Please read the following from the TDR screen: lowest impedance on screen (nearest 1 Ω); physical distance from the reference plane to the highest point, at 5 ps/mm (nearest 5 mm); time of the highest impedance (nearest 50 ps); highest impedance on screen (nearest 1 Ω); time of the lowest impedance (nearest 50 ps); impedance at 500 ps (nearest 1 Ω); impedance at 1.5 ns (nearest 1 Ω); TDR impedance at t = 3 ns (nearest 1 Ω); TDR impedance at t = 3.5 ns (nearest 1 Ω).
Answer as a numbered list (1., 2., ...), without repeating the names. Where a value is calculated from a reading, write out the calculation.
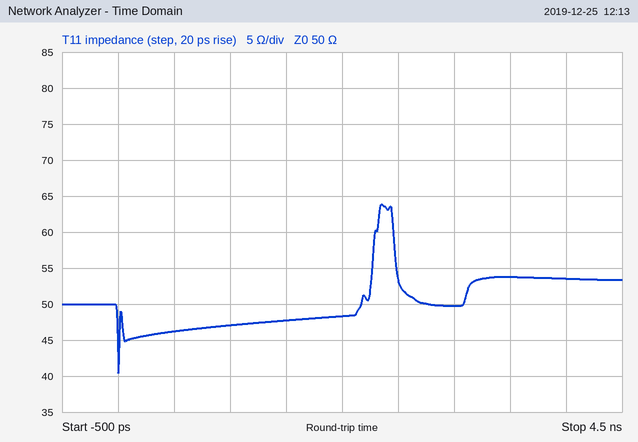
1. 40 Ω
2. 2.35 ns / 2 / 5 ps/mm ≈ 235 mm
3. 2.35 ns
4. 64 Ω
5. 0 ps
6. 46 Ω
7. 48 Ω
8. 50 Ω
9. 54 Ω
